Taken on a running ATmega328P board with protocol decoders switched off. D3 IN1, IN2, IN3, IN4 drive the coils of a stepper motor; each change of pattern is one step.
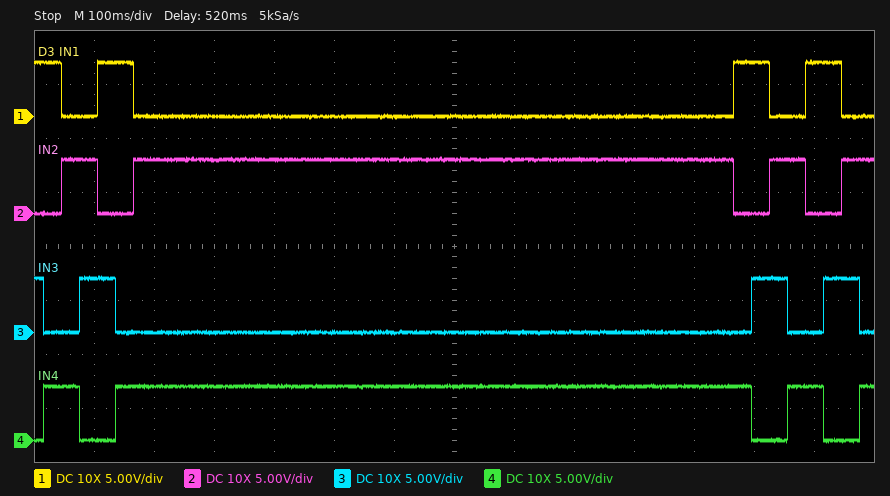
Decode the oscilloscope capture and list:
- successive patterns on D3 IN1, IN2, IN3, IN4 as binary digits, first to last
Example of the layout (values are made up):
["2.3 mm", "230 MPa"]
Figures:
["1010 1001 0101 0110 1010 1001 0101 1001 1010 0110 0101 1001 1010 0110 0101"]
